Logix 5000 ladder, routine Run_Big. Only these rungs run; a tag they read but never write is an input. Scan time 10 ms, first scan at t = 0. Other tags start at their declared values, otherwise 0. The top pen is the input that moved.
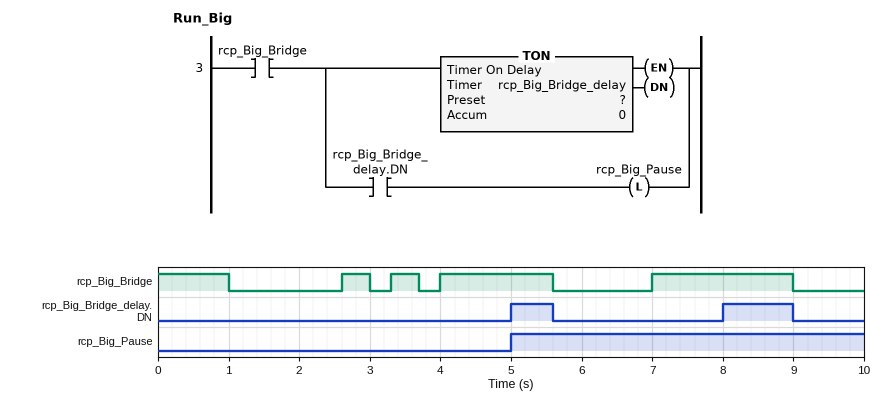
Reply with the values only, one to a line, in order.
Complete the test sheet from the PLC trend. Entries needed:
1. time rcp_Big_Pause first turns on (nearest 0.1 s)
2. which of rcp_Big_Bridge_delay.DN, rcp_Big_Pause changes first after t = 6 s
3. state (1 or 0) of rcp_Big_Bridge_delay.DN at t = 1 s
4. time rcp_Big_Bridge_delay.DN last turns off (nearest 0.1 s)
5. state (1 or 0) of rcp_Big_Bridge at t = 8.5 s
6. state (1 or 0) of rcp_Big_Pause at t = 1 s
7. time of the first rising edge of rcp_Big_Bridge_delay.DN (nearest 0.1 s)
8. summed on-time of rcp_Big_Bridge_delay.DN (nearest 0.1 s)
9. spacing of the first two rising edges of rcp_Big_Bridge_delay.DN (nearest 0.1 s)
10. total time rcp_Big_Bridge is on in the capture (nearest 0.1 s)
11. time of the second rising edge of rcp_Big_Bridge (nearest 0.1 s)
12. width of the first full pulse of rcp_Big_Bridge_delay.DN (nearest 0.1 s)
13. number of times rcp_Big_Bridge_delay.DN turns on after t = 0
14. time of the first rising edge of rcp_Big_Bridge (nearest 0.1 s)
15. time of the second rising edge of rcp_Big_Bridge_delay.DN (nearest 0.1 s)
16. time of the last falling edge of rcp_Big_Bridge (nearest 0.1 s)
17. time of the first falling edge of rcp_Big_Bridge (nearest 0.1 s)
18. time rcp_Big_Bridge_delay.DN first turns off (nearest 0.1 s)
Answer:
5.0 s
rcp_Big_Bridge_delay.DN
0
9.0 s
1
0
5.0 s
1.6 s
3.0 s
5.4 s
3.3 s
0.6 s
2
2.6 s
8.0 s
9.0 s
1.0 s
5.6 s
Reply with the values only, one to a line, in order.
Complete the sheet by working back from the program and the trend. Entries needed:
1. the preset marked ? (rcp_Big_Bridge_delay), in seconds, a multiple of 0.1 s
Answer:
1.0 s
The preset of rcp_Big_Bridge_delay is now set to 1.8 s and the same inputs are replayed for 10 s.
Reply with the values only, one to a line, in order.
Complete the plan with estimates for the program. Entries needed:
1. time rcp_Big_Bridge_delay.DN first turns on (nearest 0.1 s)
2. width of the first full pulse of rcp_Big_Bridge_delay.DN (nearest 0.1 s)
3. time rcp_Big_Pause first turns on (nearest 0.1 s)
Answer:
8.8 s
0.2 s
8.8 s
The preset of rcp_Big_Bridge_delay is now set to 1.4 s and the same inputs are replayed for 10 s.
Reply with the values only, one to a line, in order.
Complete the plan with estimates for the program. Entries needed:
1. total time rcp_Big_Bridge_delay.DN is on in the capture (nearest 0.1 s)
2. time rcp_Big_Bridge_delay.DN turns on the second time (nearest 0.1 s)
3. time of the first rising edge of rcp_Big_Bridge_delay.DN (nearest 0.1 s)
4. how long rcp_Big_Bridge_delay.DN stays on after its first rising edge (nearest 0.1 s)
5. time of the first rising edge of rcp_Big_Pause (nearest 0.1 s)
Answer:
0.8 s
8.4 s
5.4 s
0.2 s
5.4 s
